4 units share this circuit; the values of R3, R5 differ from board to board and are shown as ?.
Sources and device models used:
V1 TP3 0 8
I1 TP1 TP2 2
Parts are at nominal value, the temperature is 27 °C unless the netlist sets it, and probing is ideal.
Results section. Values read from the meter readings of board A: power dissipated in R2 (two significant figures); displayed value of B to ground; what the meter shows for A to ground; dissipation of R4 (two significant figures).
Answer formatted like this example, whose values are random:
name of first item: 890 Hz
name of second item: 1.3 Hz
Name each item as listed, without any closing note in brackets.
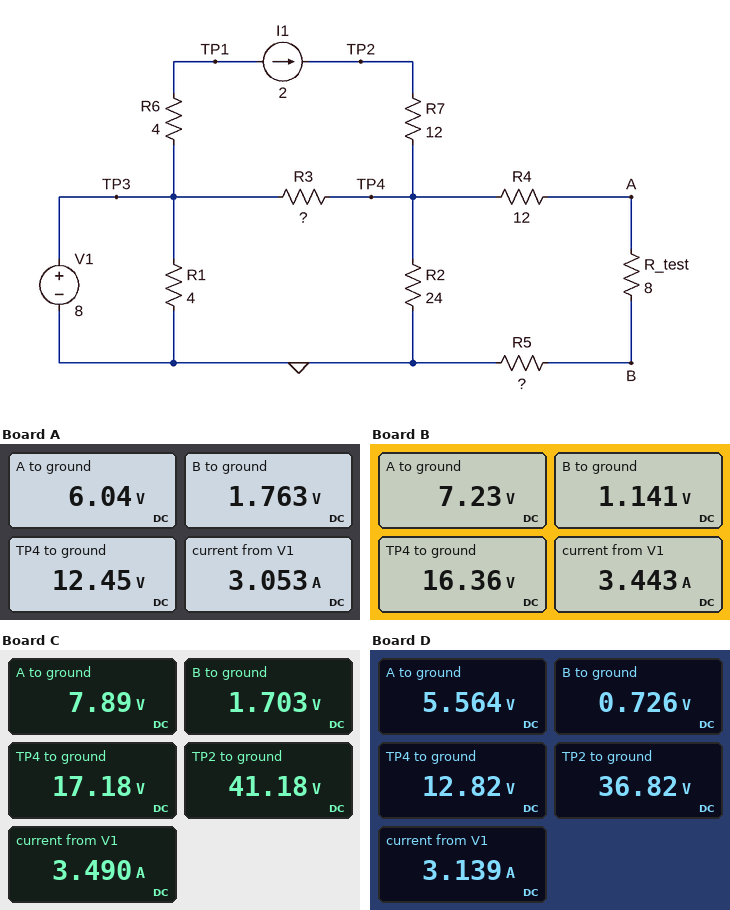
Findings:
power dissipated in R2: 6.5 W
displayed value of B to ground: 1.763 V
what the meter shows for A to ground: 6.04 V
dissipation of R4: 3.4 W
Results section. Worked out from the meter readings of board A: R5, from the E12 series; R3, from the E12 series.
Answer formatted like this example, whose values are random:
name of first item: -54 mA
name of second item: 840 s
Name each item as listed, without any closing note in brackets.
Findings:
R5, from the E12 series: 3.3 Ω
R3, from the E12 series: 4.7 Ω
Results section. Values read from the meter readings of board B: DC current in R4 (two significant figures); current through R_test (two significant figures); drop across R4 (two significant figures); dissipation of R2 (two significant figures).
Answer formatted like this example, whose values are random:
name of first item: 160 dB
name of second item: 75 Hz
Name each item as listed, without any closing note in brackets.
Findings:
DC current in R4: 760 mA
current through R_test: 760 mA
drop across R4: 9.1 V
dissipation of R2: 11 W
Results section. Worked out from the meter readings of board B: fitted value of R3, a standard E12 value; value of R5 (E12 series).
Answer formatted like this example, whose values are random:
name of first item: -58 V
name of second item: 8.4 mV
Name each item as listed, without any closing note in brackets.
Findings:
fitted value of R3, a standard E12 value: 15 Ω
value of R5: 1.5 Ω
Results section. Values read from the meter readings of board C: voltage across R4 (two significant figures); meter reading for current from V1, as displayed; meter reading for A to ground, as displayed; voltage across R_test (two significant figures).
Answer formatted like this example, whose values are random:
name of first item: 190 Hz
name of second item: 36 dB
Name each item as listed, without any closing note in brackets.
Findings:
voltage across R4: 9.3 V
meter reading for current from V1, as displayed: 3.490 A
meter reading for A to ground, as displayed: 7.89 V
voltage across R_test: 6.2 V
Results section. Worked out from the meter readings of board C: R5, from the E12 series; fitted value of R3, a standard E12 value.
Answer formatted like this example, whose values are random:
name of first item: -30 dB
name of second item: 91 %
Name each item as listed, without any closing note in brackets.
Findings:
R5, from the E12 series: 2.2 Ω
fitted value of R3, a standard E12 value: 18 Ω
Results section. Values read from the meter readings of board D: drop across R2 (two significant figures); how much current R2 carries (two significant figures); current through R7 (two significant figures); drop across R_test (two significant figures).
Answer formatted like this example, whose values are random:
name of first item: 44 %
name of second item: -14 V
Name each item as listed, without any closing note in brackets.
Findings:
drop across R2: 13 V
how much current R2 carries: 530 mA
current through R7: 2.0 A
drop across R_test: 4.8 V
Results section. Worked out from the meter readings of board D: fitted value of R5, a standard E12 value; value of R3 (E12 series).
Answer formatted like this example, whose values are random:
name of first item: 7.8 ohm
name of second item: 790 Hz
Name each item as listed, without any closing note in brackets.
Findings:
fitted value of R5, a standard E12 value: 1.2 Ω
value of R3: 5.6 Ω
